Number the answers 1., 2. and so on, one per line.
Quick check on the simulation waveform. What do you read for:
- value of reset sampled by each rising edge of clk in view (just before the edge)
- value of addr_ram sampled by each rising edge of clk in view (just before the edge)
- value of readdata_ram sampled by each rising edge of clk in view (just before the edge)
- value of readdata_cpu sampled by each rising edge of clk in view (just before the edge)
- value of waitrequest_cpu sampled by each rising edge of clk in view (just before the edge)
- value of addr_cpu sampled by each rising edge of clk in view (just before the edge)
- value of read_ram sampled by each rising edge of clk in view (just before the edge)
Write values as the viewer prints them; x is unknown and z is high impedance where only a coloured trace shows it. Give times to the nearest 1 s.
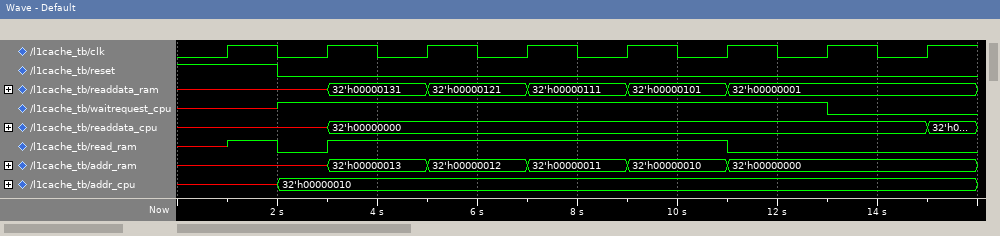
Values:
1. 1 0 0 0 0 0 0 0
2. x, x, 32'h00000013, 32'h00000012, 32'h00000011, 32'h00000010, 32'h00000000, 32'h00000000
3. x, x, 32'h00000131, 32'h00000121, 32'h00000111, 32'h00000101, 32'h00000001, 32'h00000001
4. x, x, 32'h00000000, 32'h00000000, 32'h00000000, 32'h00000000, 32'h00000000, 32'h00000000
5. x 1 1 1 1 1 1 0
6. x, 32'h00000010, 32'h00000010, 32'h00000010, 32'h00000010, 32'h00000010, 32'h00000010, 32'h00000010
7. x 0 1 1 1 1 0 0
